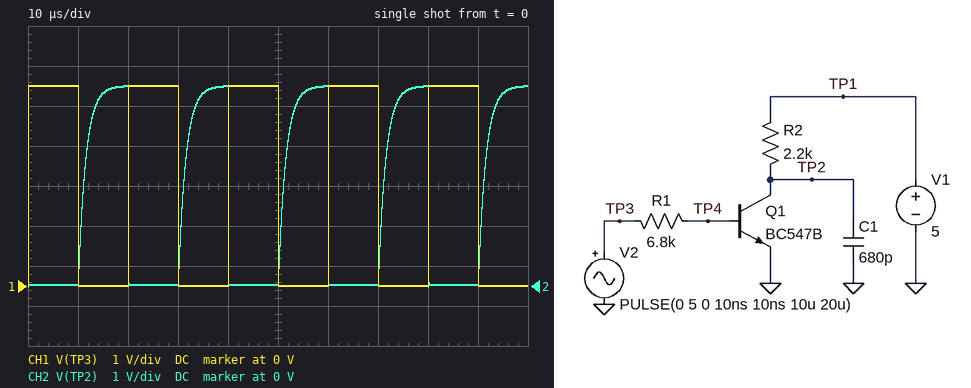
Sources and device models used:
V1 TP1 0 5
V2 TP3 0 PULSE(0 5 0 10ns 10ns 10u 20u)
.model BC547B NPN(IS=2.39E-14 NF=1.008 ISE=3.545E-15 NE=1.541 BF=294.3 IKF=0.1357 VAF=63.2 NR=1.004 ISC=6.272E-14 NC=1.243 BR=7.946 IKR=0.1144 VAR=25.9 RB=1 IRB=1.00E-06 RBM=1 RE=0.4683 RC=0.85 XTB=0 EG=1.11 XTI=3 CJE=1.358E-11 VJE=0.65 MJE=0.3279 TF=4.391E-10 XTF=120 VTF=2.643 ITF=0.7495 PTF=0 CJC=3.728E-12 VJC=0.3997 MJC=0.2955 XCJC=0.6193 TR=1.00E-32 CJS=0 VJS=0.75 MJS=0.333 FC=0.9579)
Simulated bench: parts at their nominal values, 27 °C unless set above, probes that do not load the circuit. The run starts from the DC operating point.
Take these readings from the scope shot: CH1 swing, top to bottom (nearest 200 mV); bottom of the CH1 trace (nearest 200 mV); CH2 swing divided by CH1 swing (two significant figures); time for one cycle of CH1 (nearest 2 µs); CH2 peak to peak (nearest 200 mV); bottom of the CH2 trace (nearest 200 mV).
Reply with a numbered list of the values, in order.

1. 5.0 V
2. 0 V
3. 1.0
4. 20 µs
5. 5.0 V
6. 0 V
